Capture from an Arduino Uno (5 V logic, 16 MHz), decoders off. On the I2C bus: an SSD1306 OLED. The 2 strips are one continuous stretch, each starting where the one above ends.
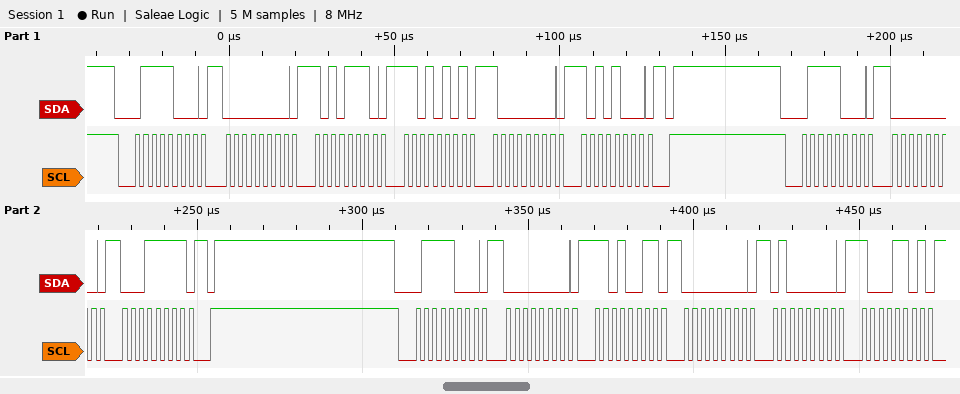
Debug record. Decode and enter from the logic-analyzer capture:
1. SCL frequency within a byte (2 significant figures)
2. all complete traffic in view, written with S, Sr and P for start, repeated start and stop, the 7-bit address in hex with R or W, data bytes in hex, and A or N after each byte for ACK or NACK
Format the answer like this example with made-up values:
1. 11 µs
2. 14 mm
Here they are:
1. 400 kHz
2. S 3CW A 00 A AE A D5 A 80 A A8 A P S 3CW A 00 A 1F A P S 3CW A 00 A D3 A 00 A 40 A 8D A
